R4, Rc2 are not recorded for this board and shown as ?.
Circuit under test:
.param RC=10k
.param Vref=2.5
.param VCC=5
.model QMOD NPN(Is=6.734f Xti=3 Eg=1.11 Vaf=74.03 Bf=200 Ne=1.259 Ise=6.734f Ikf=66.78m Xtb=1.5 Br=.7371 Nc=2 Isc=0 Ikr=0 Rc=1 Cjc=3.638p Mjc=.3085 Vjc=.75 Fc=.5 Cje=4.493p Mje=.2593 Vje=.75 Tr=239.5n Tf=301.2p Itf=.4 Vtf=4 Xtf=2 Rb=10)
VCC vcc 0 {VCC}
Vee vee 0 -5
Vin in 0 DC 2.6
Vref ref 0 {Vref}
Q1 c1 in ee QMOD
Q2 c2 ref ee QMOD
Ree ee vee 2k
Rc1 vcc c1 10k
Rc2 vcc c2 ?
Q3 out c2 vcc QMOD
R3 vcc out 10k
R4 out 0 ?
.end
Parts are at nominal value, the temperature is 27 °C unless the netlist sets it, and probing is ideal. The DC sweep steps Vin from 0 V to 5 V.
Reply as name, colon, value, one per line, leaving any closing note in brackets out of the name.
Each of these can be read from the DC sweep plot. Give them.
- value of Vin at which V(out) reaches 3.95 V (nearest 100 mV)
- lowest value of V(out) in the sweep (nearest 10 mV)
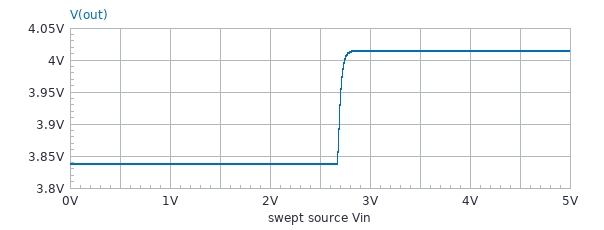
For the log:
value of Vin at which V(out) reaches 3.95 V: 2.7 V
lowest value of V(out) in the sweep: 3.84 V
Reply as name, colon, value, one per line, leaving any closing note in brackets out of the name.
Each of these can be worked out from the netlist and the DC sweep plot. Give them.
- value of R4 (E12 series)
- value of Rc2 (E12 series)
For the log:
value of R4: 33 kΩ
value of Rc2: 33 kΩ
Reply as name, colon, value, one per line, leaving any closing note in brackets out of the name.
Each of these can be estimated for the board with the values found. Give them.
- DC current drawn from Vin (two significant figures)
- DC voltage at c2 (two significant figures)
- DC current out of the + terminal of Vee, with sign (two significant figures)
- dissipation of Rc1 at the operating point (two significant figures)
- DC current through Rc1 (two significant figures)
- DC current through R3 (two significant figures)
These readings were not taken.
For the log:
DC current drawn from Vin: 2.9 mA
DC voltage at c2: 1.9 V
DC current out of the + terminal of Vee, with sign: -3.4 mA
dissipation of Rc1 at the operating point: 970 µW
DC current through Rc1: 310 µA
DC current through R3: 120 µA
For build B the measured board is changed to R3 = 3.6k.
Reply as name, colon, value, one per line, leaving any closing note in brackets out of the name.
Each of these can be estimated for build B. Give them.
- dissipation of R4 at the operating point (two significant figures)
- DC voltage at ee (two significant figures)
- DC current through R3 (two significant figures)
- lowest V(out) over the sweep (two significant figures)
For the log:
dissipation of R4 at the operating point: 620 µW
DC voltage at ee: 1.9 V
DC current through R3: 140 µA
lowest V(out) over the sweep: 4.5 V
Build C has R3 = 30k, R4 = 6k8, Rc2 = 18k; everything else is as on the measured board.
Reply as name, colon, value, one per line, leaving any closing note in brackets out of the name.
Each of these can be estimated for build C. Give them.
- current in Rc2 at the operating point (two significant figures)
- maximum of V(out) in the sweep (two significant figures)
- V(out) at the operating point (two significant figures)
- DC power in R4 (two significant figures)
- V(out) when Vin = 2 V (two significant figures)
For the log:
current in Rc2 at the operating point: 170 µA
maximum of V(out) in the sweep: 2.1 V
V(out) at the operating point: 1.3 V
DC power in R4: 260 µW
V(out) when Vin = 2 V: 1.2 V
